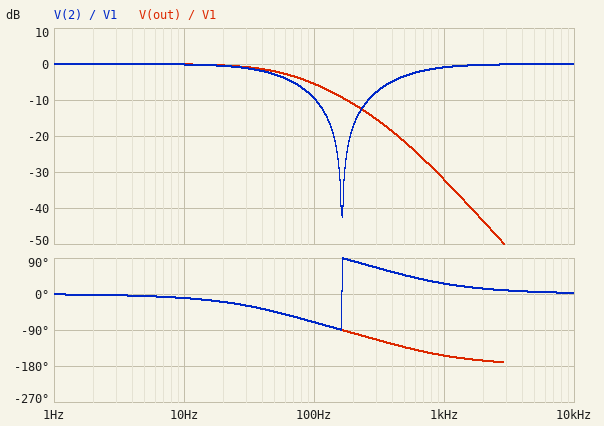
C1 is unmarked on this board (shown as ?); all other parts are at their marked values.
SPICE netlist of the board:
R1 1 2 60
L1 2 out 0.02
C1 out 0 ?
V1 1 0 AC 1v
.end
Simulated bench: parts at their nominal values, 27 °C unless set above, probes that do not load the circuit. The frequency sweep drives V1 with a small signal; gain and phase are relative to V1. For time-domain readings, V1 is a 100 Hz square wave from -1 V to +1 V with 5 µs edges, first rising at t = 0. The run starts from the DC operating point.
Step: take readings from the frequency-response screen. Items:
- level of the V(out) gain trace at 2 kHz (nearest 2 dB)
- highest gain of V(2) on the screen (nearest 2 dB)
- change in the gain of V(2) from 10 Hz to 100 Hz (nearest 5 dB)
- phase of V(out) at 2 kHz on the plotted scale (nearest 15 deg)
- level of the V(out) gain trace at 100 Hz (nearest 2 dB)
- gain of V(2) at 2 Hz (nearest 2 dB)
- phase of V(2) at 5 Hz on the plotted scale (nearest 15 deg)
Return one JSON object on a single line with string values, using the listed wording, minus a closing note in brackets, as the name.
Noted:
{"level of the V(out) gain trace at 2 kHz": "-44 dB", "highest gain of V(2) on the screen": "0 dB", "change in the gain of V(2) from 10 Hz to 100 Hz": "-10 dB", "phase of V(out) at 2 kHz on the plotted scale": "-165 deg", "level of the V(out) gain trace at 100 Hz": "-6 dB", "gain of V(2) at 2 Hz": "0 dB", "phase of V(2) at 5 Hz on the plotted scale": "0 deg"}
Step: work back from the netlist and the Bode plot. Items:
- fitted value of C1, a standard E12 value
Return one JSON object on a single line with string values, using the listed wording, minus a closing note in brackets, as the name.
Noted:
{"fitted value of C1, a standard E12 value": "47 µF"}
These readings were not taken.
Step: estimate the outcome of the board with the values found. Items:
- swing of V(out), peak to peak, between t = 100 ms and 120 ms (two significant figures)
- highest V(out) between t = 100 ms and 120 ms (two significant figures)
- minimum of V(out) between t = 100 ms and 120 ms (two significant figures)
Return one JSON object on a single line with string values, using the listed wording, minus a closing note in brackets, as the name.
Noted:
{"swing of V(out), peak to peak, between t = 100 ms and 120 ms": "1.5 V", "highest V(out) between t = 100 ms and 120 ms": "730 mV", "minimum of V(out) between t = 100 ms and 120 ms": "-730 mV"}
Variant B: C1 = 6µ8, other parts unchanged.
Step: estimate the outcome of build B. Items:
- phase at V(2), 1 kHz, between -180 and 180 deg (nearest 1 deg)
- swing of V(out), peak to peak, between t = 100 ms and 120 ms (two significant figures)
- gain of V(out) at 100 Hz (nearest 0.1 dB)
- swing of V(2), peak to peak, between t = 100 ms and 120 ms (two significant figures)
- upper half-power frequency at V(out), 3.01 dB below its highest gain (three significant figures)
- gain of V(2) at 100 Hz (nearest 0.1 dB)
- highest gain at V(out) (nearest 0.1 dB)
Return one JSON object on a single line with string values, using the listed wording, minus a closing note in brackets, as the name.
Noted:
{"phase at V(2), 1 kHz, between -180 and 180 deg": "30 deg", "swing of V(out), peak to peak, between t = 100 ms and 120 ms": "2.5 V", "gain of V(out) at 100 Hz": "0.2 dB", "swing of V(2), peak to peak, between t = 100 ms and 120 ms": "2.3 V", "upper half-power frequency at V(out), 3.01 dB below its highest gain": "494 Hz", "gain of V(2) at 100 Hz": "-0.3 dB", "highest gain at V(out)": "0.7 dB"}
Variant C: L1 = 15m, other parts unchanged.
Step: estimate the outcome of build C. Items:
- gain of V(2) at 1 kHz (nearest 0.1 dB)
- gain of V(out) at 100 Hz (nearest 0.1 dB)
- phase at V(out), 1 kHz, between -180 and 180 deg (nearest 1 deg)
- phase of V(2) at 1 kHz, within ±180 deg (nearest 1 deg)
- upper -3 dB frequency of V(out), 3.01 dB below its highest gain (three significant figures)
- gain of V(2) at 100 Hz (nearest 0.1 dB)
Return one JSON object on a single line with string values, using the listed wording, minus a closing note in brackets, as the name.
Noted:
{"gain of V(2) at 1 kHz": "-1.6 dB", "gain of V(out) at 100 Hz": "-5.6 dB", "phase at V(out), 1 kHz, between -180 and 180 deg": "-147 deg", "phase of V(2) at 1 kHz, within ±180 deg": "33 deg", "upper -3 dB frequency of V(out), 3.01 dB below its highest gain": "61.9 Hz", "gain of V(2) at 100 Hz": "-8.5 dB"}
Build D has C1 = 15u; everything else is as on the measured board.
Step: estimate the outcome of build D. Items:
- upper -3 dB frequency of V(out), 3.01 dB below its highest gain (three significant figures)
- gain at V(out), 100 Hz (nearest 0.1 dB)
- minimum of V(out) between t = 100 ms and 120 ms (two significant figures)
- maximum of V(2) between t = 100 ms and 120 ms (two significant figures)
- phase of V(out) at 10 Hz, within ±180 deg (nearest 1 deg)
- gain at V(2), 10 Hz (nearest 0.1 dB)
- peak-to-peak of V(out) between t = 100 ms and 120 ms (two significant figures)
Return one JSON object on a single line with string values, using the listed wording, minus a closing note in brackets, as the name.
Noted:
{"upper -3 dB frequency of V(out), 3.01 dB below its highest gain": "245 Hz", "gain at V(out), 100 Hz": "-0.4 dB", "minimum of V(out) between t = 100 ms and 120 ms": "-1.0 V", "maximum of V(2) between t = 100 ms and 120 ms": "1.0 V", "phase of V(out) at 10 Hz, within ±180 deg": "-3 deg", "gain at V(2), 10 Hz": "0 dB", "peak-to-peak of V(out) between t = 100 ms and 120 ms": "2.0 V"}
